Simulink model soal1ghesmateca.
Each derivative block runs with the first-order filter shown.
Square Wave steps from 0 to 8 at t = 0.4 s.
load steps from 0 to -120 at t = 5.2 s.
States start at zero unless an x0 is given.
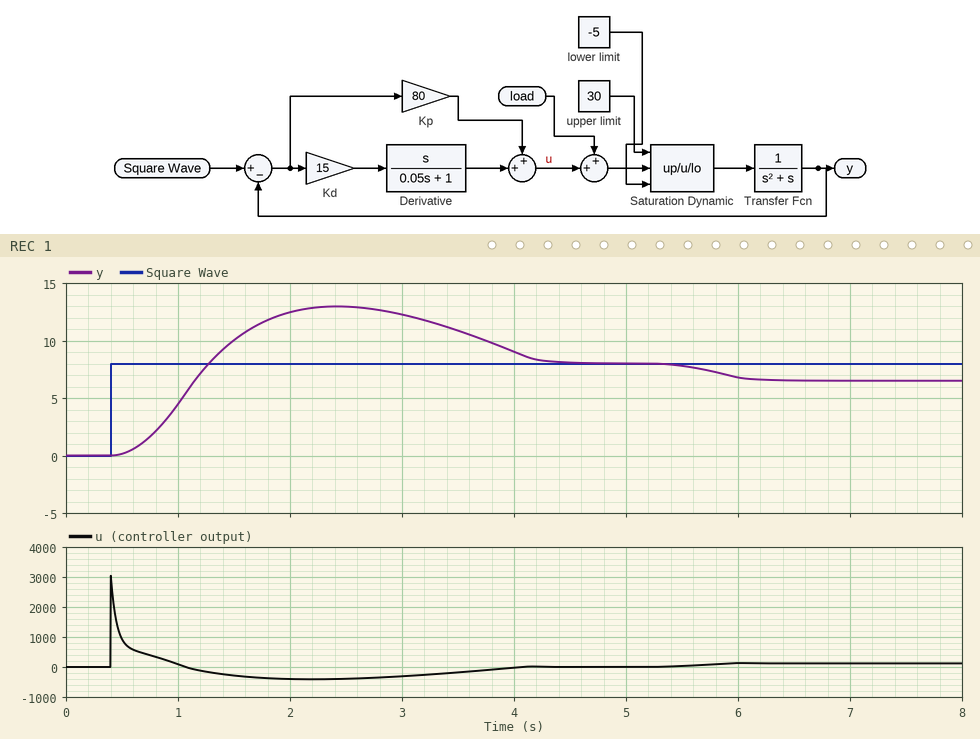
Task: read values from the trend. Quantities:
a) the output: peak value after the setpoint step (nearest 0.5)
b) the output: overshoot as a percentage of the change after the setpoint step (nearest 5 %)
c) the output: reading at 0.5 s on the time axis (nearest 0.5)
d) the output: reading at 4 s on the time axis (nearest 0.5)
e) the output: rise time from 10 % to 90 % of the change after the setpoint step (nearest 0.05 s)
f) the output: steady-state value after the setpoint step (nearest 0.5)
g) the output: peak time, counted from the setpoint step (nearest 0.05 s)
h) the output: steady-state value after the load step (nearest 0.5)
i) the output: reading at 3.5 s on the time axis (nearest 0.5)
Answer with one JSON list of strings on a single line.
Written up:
["13.0", "60 %", "0.0", "9.0", "0.55 s", "8.0", "2.00 s", "6.5", "11.0"]
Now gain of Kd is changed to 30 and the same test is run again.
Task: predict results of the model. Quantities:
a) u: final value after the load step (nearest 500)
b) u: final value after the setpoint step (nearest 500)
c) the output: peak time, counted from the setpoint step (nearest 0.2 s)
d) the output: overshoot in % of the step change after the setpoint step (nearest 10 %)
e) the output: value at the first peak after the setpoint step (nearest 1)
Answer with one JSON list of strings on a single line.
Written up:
["0", "0", "1.8 s", "20 %", "10"]
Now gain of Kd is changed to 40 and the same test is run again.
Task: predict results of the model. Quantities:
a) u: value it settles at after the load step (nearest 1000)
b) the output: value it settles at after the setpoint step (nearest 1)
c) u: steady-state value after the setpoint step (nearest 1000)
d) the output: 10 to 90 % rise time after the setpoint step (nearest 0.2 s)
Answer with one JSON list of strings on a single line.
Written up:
["0", "8", "0", "0.8 s"]
